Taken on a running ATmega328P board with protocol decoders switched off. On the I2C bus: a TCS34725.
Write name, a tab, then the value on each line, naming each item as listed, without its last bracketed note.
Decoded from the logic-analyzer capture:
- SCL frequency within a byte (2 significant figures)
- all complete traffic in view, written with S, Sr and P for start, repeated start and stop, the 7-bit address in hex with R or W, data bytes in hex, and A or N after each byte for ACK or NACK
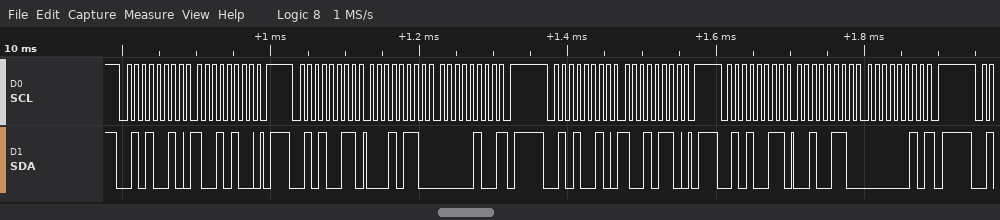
SCL frequency within a byte	100 kHz
all complete traffic in view, written with S, Sr and P for start, repeated start and stop, the 7-bit address in hex with R or W, data bytes in hex, and A or N after each byte for ACK or NACK	S 29W A 94 A P S 29R A 16 A 04 N P S 29W A 96 A P S 29R A 26 A 02 N P
